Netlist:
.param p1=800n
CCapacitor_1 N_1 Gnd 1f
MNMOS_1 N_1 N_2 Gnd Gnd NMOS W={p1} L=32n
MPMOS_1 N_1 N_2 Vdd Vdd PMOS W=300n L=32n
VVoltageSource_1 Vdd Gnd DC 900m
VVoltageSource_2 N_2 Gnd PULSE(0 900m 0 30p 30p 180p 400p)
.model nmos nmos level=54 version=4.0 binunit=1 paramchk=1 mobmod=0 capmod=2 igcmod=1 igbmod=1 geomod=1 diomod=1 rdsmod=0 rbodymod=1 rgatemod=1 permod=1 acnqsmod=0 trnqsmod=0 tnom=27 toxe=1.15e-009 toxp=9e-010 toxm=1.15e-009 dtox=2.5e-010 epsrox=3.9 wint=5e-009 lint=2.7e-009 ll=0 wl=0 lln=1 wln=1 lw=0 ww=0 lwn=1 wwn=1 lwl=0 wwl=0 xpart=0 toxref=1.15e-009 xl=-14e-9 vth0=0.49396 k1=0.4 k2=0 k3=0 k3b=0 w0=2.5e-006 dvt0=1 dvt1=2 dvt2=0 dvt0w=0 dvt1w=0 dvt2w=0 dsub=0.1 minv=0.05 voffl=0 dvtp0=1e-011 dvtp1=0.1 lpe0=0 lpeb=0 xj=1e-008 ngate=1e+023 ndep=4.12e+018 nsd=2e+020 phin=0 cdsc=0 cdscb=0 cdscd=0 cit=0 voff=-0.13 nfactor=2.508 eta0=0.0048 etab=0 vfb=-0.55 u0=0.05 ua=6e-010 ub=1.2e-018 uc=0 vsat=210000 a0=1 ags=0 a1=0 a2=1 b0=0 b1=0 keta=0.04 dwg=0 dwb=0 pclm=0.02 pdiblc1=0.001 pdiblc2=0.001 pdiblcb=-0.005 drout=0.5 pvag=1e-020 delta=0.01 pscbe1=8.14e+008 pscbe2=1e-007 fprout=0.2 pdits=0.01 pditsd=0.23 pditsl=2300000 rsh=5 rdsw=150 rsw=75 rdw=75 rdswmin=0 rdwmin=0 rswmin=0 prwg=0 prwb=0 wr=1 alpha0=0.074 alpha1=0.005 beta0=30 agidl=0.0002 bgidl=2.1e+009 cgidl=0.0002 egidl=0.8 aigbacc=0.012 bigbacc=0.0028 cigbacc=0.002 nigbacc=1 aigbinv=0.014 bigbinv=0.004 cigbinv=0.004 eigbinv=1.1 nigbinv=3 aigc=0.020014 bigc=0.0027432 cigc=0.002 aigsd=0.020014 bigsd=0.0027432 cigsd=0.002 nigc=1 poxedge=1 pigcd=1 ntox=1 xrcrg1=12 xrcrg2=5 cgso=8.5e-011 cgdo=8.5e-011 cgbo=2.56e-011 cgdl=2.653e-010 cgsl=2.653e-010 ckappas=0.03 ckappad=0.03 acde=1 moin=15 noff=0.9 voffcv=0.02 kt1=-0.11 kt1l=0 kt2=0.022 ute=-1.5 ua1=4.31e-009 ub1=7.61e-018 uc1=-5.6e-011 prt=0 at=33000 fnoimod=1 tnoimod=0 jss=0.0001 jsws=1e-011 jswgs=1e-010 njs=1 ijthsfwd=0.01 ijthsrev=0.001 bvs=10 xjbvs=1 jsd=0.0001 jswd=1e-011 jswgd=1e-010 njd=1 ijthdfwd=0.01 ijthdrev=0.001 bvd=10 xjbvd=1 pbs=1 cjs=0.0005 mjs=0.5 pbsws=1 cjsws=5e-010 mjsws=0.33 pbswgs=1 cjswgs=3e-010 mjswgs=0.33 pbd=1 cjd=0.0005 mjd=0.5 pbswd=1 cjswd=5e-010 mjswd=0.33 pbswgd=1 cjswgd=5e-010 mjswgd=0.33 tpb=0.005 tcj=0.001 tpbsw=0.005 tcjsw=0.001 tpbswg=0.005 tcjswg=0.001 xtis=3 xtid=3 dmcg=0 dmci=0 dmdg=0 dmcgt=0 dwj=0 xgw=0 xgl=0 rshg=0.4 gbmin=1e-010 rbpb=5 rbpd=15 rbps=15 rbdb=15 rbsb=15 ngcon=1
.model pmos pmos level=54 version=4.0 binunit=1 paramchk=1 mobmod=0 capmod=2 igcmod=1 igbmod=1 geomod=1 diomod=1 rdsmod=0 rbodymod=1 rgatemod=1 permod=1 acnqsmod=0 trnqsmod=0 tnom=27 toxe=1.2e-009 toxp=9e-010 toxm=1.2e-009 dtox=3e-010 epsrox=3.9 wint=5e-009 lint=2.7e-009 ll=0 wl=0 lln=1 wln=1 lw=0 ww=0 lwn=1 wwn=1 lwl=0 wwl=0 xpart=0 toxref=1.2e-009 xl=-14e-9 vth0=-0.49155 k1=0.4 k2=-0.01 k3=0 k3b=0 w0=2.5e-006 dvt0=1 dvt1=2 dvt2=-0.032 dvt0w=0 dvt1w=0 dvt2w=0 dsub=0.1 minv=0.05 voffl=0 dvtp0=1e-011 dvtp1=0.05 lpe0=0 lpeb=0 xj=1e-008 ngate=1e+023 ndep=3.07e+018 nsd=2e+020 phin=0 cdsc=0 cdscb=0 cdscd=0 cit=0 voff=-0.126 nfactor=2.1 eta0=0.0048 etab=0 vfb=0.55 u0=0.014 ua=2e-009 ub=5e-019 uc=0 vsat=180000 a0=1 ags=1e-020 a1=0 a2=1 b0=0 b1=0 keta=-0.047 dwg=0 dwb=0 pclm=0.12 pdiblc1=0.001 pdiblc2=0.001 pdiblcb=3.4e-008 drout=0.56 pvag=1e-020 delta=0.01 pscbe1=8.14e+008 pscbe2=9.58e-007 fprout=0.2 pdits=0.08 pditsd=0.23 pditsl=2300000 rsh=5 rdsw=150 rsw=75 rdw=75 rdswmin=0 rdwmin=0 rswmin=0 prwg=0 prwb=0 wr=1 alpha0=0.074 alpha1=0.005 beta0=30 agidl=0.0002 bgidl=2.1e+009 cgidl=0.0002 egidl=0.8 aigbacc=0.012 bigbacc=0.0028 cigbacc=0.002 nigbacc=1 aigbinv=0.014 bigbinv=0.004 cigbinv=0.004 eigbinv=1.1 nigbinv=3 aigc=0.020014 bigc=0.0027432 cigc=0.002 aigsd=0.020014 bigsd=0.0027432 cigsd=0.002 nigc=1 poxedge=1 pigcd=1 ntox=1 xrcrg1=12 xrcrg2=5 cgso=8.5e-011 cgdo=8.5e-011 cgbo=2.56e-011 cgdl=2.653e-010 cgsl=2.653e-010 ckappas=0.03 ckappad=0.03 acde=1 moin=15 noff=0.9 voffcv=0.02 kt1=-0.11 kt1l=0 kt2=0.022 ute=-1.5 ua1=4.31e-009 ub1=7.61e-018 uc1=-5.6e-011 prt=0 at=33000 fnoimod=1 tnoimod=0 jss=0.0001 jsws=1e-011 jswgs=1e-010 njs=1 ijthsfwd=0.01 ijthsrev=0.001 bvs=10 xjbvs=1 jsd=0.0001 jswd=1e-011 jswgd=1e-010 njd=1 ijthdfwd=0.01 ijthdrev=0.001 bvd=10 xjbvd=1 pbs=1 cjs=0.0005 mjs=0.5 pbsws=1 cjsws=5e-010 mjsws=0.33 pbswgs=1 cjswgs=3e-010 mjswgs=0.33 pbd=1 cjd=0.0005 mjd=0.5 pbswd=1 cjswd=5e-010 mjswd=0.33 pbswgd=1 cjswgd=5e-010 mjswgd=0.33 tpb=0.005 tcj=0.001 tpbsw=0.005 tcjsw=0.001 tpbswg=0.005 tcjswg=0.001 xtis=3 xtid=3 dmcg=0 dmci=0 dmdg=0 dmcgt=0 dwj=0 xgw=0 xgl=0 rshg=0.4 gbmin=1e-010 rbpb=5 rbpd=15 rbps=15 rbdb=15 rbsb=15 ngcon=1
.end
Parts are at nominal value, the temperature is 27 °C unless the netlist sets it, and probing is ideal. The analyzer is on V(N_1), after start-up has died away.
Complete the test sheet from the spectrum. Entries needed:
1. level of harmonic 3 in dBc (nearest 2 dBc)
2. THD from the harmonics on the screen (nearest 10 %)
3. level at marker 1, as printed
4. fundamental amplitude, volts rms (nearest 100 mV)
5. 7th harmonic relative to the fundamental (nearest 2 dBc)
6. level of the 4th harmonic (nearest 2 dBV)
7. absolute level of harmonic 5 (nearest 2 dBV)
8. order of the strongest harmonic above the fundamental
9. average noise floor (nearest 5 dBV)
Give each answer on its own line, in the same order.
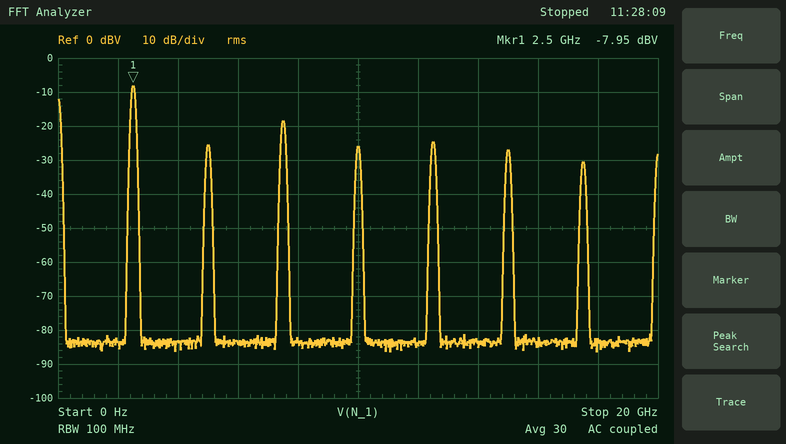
-10 dBc
40 %
-7.95 dBV
400 mV
-22 dBc
-26 dBV
-24 dBV
3
-85 dBV
